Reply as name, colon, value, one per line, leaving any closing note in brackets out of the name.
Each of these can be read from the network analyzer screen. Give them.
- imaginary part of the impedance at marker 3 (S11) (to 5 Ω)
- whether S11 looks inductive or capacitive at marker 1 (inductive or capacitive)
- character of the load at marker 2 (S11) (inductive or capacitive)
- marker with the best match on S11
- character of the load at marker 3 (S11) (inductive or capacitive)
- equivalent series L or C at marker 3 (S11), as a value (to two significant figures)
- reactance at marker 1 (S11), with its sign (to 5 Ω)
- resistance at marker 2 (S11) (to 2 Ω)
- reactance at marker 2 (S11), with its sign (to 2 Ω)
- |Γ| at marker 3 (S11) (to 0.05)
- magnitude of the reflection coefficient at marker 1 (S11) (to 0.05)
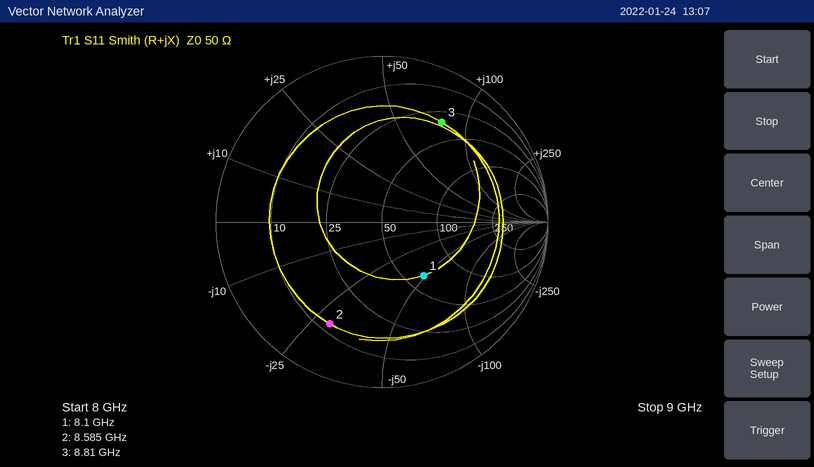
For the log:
imaginary part of the impedance at marker 3 (S11): +80 Ω
whether S11 looks inductive or capacitive at marker 1: capacitive
character of the load at marker 2 (S11): capacitive
marker with the best match on S11: marker 1
character of the load at marker 3 (S11): inductive
equivalent series L or C at marker 3 (S11), as a value: 1.4 nH
reactance at marker 1 (S11), with its sign: -50 Ω
resistance at marker 2 (S11): 12 Ω
reactance at marker 2 (S11), with its sign: -30 Ω
|Γ| at marker 3 (S11): 0.70
magnitude of the reflection coefficient at marker 1 (S11): 0.40
